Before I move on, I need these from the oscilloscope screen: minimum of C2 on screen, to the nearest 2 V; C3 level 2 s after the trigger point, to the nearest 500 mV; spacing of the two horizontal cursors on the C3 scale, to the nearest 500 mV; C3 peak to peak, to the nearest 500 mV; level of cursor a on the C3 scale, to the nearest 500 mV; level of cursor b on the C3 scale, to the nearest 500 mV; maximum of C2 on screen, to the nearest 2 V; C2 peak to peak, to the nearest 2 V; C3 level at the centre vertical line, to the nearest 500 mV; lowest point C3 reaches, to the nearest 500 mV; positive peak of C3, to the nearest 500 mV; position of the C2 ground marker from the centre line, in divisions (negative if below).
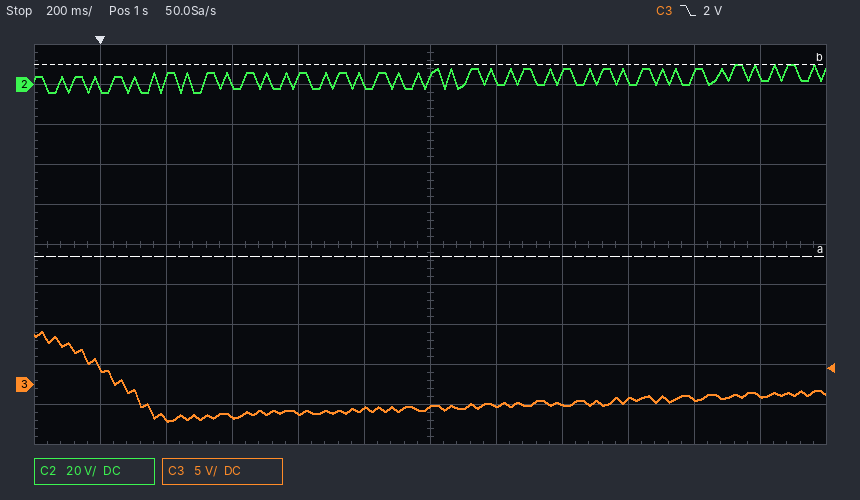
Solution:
-4 V
-1.5 V
24.0 V
11.0 V
16.0 V
40.0 V
10 V
14 V
-3.0 V
-4.5 V
6.5 V
+4.0 div
